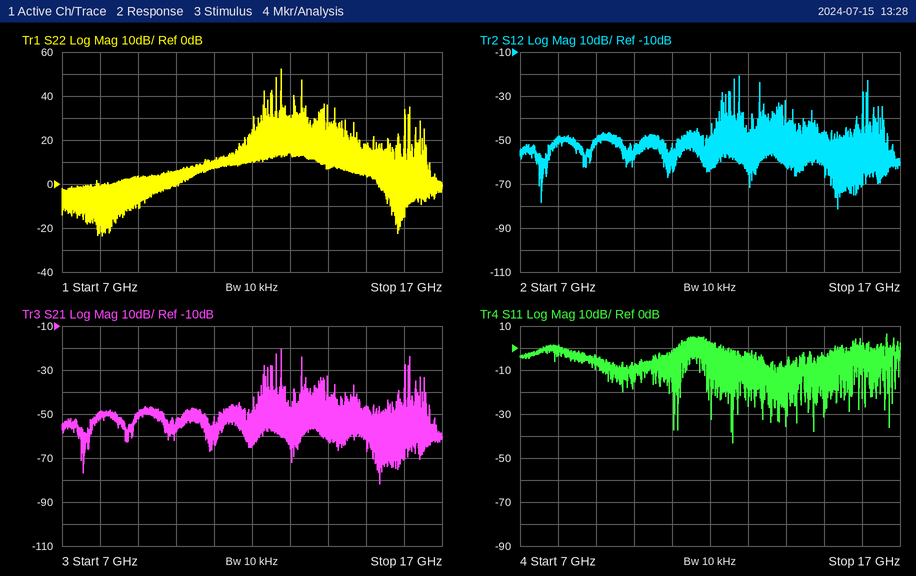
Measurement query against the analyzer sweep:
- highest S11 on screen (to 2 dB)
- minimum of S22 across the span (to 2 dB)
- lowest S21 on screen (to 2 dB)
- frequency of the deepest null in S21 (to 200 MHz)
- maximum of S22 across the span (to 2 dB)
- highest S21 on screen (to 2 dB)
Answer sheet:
6 dB
-24 dB
-82 dB
15.4 GHz
52 dB
-20 dB
